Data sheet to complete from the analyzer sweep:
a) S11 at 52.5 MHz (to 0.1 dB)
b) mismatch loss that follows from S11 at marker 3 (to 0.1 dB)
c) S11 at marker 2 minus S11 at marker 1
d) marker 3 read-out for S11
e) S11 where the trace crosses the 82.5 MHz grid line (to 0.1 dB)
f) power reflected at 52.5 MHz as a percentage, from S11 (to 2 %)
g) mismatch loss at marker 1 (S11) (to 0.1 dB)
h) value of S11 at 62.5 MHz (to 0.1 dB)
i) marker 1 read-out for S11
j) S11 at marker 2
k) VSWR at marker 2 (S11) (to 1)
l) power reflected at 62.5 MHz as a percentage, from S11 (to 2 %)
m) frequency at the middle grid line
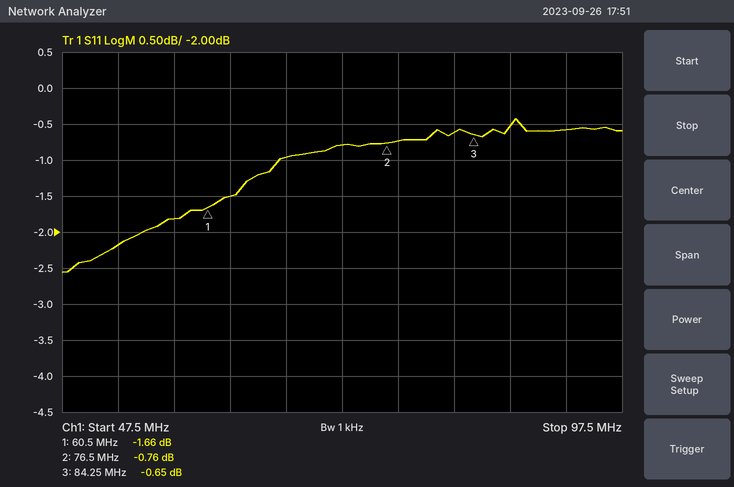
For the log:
-2.2 dB
8.6 dB
0.90 dB
-0.65 dB
-0.6 dB
60 %
5.0 dB
-1.5 dB
-1.66 dB
-0.76 dB
23
70 %
72.5 MHz
